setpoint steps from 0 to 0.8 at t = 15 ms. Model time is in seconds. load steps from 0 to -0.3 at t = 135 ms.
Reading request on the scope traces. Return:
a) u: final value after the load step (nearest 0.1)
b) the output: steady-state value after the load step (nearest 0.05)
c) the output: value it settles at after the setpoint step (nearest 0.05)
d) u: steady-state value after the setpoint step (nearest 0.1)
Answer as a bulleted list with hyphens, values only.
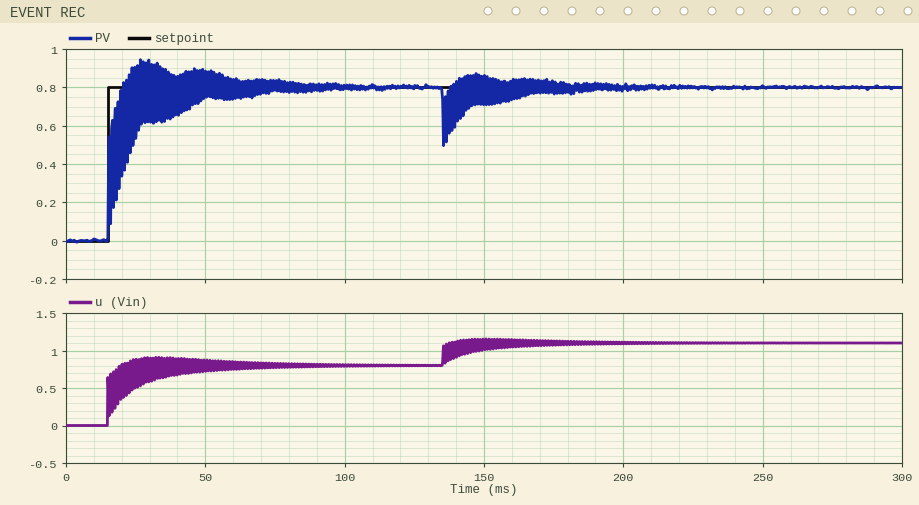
- 1.1
- 0.80
- 0.80
- 0.8
